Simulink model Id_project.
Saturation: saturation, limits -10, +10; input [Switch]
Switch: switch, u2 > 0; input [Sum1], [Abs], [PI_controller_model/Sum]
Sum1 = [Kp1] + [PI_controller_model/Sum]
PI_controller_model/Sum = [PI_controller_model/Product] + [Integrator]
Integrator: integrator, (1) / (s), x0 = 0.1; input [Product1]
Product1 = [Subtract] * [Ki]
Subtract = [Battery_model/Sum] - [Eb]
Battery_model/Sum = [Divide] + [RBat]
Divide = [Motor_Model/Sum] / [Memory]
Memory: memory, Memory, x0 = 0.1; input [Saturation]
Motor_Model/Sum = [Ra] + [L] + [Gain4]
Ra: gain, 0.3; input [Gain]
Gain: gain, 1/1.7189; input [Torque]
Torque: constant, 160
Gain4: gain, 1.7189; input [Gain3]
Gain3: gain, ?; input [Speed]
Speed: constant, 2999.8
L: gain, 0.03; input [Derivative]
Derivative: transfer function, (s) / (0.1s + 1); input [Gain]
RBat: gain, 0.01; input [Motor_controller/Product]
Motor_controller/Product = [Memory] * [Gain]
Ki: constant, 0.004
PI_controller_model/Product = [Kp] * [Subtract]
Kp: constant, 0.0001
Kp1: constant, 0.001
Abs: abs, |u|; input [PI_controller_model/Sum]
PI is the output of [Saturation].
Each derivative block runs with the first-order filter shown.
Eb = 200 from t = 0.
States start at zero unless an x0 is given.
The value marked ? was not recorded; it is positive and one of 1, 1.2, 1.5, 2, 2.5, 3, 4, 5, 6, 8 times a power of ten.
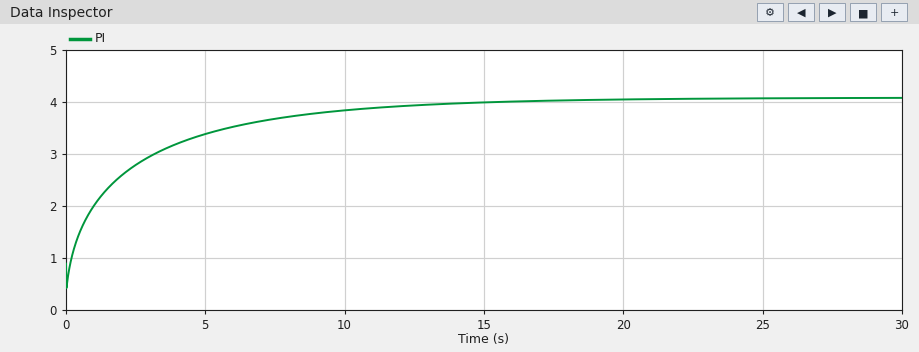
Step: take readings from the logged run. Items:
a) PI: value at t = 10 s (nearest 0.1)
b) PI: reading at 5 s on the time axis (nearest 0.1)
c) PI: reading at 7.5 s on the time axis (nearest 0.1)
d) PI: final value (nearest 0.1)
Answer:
3.8
3.4
3.7
4.1
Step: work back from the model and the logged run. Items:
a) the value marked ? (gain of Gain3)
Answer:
0.15
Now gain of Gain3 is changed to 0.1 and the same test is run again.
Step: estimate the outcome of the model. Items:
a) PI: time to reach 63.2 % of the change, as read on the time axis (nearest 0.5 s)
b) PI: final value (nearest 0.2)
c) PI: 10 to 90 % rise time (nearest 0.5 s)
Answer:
2.0 s
2.8
5.5 s
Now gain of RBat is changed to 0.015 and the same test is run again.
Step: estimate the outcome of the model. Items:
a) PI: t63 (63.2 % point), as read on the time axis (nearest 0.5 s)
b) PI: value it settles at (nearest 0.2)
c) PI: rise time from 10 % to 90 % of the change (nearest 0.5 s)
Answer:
3.0 s
4.2
8.5 s
